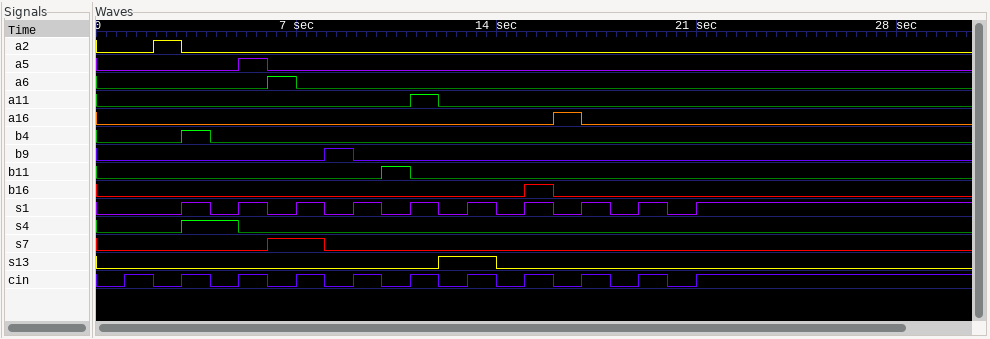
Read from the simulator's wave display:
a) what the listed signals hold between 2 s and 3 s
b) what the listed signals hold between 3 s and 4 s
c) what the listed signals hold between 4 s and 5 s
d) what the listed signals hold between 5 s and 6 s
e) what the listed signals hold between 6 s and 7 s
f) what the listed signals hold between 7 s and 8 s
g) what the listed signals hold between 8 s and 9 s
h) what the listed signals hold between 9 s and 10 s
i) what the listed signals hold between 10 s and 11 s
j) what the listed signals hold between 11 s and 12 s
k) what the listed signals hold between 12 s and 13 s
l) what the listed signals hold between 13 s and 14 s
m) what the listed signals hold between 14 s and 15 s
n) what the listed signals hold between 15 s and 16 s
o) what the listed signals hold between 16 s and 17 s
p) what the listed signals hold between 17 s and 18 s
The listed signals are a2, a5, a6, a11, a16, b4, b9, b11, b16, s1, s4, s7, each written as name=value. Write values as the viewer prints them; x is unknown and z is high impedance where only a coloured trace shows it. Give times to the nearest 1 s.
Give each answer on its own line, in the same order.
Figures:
a2=1, a5=0, a6=0, a11=0, a16=0, b4=0, b9=0, b11=0, b16=0, s1=0, s4=0, s7=0
a2=0, a5=0, a6=0, a11=0, a16=0, b4=1, b9=0, b11=0, b16=0, s1=1, s4=1, s7=0
a2=0, a5=0, a6=0, a11=0, a16=0, b4=0, b9=0, b11=0, b16=0, s1=0, s4=1, s7=0
a2=0, a5=1, a6=0, a11=0, a16=0, b4=0, b9=0, b11=0, b16=0, s1=1, s4=0, s7=0
a2=0, a5=0, a6=1, a11=0, a16=0, b4=0, b9=0, b11=0, b16=0, s1=0, s4=0, s7=1
a2=0, a5=0, a6=0, a11=0, a16=0, b4=0, b9=0, b11=0, b16=0, s1=1, s4=0, s7=1
a2=0, a5=0, a6=0, a11=0, a16=0, b4=0, b9=1, b11=0, b16=0, s1=0, s4=0, s7=0
a2=0, a5=0, a6=0, a11=0, a16=0, b4=0, b9=0, b11=0, b16=0, s1=1, s4=0, s7=0
a2=0, a5=0, a6=0, a11=0, a16=0, b4=0, b9=0, b11=1, b16=0, s1=0, s4=0, s7=0
a2=0, a5=0, a6=0, a11=1, a16=0, b4=0, b9=0, b11=0, b16=0, s1=1, s4=0, s7=0
a2=0, a5=0, a6=0, a11=0, a16=0, b4=0, b9=0, b11=0, b16=0, s1=0, s4=0, s7=0
a2=0, a5=0, a6=0, a11=0, a16=0, b4=0, b9=0, b11=0, b16=0, s1=1, s4=0, s7=0
a2=0, a5=0, a6=0, a11=0, a16=0, b4=0, b9=0, b11=0, b16=0, s1=0, s4=0, s7=0
a2=0, a5=0, a6=0, a11=0, a16=0, b4=0, b9=0, b11=0, b16=1, s1=1, s4=0, s7=0
a2=0, a5=0, a6=0, a11=0, a16=1, b4=0, b9=0, b11=0, b16=0, s1=0, s4=0, s7=0
a2=0, a5=0, a6=0, a11=0, a16=0, b4=0, b9=0, b11=0, b16=0, s1=1, s4=0, s7=0
